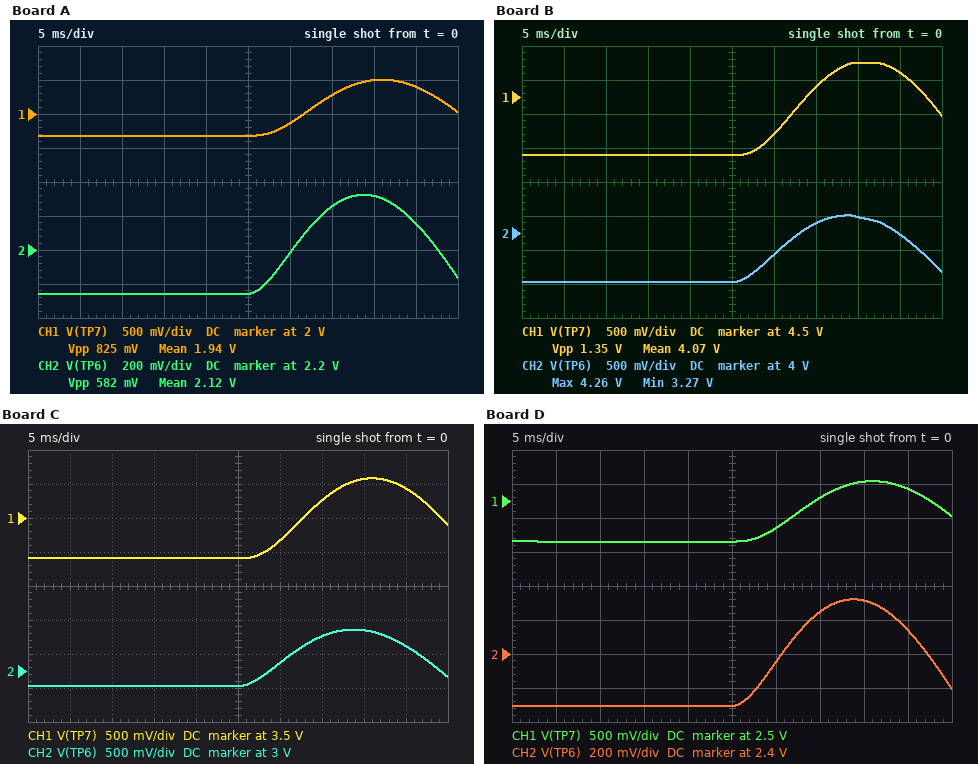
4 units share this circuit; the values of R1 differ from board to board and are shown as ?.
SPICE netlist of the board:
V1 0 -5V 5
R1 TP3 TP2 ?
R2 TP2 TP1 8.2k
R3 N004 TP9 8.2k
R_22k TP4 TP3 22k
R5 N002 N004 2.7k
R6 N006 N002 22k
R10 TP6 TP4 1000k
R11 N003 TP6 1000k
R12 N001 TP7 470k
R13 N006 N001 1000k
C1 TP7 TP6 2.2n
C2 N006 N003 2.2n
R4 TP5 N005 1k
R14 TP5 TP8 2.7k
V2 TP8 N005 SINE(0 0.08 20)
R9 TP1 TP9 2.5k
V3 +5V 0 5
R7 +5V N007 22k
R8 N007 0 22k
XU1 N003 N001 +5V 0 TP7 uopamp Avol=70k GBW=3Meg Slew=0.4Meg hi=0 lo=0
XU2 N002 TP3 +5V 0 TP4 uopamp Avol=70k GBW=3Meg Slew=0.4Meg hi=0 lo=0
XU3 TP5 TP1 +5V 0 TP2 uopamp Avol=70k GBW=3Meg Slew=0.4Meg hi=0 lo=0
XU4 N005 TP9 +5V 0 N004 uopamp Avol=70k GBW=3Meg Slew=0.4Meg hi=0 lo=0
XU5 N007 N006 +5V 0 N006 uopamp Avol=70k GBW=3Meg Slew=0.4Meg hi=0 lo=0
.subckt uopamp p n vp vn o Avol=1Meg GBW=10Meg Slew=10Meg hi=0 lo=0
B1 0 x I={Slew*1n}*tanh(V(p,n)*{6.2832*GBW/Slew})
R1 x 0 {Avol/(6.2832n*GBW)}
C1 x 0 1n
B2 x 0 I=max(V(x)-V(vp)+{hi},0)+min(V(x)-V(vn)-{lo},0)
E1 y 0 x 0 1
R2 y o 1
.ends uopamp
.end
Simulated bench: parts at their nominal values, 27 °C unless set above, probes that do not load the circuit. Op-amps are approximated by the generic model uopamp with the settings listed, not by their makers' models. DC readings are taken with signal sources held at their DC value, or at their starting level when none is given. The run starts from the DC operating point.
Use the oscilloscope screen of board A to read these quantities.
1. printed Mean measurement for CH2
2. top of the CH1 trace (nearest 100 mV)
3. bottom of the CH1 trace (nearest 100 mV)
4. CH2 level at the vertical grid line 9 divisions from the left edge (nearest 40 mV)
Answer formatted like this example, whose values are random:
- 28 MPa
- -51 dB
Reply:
- 2.12 V
- 2.5 V
- 1.7 V
- 2.36 V
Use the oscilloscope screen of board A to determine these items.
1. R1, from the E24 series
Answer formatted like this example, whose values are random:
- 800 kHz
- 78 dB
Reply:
- 3.6 kΩ
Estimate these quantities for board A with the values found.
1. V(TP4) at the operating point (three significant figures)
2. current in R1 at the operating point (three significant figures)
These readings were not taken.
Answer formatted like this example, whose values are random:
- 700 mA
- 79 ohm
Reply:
- 1.94 V
- 75.9 µA
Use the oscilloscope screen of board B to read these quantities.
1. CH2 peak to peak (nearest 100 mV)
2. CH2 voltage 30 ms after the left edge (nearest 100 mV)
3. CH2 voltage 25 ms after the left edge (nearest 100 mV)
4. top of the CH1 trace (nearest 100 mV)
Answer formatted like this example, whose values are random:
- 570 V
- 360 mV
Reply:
- 1.0 V
- 3.7 V
- 3.3 V
- 5.0 V
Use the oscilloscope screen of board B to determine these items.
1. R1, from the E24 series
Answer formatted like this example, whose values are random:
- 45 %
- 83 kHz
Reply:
- 2 kΩ
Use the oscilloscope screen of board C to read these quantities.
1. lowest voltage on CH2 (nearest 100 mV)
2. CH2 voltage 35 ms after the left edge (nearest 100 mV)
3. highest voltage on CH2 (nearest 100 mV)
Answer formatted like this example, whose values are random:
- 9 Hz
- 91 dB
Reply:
- 2.8 V
- 3.5 V
- 3.6 V
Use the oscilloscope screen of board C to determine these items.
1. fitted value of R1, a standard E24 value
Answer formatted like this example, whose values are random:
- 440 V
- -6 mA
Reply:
- 2.4 kΩ
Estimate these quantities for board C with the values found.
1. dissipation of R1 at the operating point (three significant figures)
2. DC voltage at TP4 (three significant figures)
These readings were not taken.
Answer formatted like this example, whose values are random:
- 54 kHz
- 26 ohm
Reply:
- 31.1 µW
- 2.78 V
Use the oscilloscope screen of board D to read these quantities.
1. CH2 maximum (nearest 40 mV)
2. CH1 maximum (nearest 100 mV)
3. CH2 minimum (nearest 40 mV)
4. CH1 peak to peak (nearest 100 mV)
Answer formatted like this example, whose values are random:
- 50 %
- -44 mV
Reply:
- 2.72 V
- 2.8 V
- 2.08 V
- 900 mV
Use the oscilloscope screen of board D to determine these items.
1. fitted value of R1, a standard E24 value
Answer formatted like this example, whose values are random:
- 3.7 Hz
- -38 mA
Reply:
- 3.3 kΩ
